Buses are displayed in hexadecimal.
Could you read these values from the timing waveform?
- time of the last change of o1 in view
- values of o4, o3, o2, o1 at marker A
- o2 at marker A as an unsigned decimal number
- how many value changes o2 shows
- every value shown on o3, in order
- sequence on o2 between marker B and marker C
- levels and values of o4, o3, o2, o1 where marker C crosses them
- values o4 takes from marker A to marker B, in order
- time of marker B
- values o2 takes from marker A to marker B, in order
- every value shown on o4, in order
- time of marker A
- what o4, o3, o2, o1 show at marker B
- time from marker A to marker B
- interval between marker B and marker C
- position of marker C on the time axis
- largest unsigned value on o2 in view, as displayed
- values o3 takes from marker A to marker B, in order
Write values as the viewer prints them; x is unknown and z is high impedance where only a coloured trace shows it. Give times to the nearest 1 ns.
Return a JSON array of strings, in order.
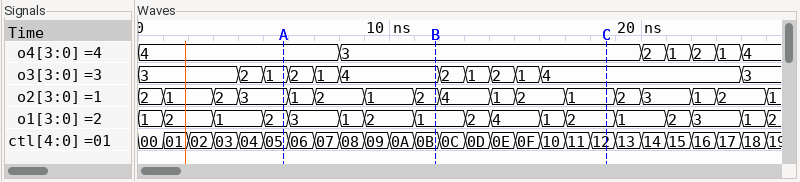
["25 ns", "o4=4, o3=1, o2=3, o1=2", "3", "16", "3, 2, 1, 2, 1, 4, 2, 1, 2, 1, 4, 3", "2, 4, 1, 2, 1", "o4=3, o3=4, o2=1, o1=2", "4, 3", "12 ns", "3, 1, 2, 1, 2", "4, 3, 2, 1, 2, 1, 4", "6 ns", "o4=3, o3=4, o2=2, o1=1", "6 ns", "7 ns", "19 ns", "4", "1, 2, 1, 4"]
